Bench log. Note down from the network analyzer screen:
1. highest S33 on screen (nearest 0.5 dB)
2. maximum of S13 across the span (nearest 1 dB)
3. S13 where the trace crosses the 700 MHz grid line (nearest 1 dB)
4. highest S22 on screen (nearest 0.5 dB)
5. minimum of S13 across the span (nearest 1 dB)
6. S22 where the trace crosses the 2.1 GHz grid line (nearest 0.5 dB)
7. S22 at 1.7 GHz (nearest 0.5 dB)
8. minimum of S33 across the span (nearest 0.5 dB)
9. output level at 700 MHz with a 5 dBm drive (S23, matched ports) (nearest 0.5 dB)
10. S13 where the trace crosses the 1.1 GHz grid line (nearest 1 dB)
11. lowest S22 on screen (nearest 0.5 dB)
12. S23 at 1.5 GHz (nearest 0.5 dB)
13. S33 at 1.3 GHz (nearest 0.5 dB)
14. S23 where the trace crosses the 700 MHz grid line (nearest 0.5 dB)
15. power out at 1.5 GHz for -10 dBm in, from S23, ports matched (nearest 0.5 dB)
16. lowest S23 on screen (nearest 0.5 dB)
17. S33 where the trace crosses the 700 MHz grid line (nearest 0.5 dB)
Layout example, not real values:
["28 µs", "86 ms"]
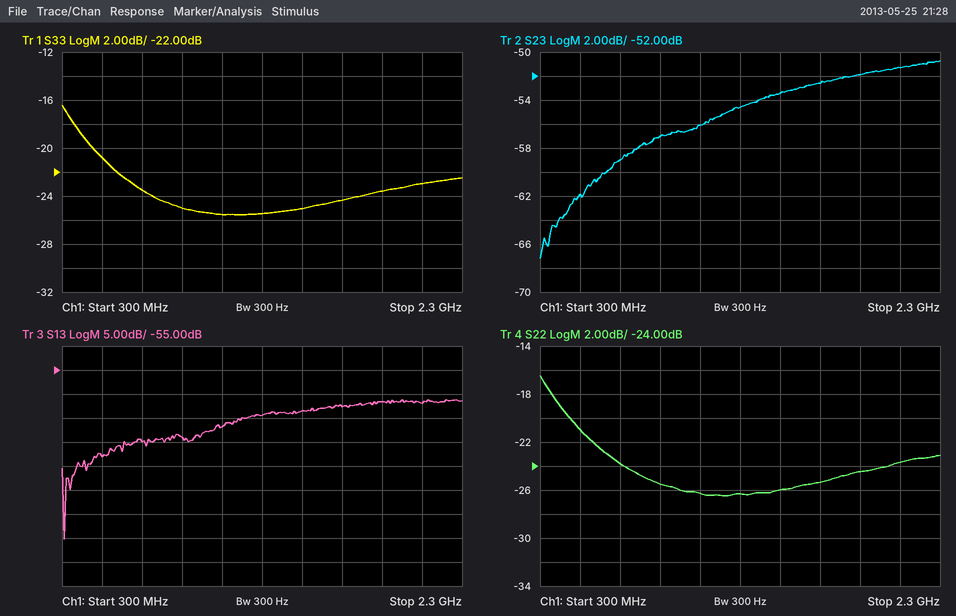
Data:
["-16.5 dB", "-61 dB", "-70 dB", "-16.5 dB", "-90 dB", "-23.5 dB", "-25.5 dB", "-25.5 dB", "-54.0 dBm", "-67 dB", "-26.5 dB", "-53.5 dB", "-25.5 dB", "-59.0 dB", "-63.5 dBm", "-67.0 dB", "-23.5 dB"]
